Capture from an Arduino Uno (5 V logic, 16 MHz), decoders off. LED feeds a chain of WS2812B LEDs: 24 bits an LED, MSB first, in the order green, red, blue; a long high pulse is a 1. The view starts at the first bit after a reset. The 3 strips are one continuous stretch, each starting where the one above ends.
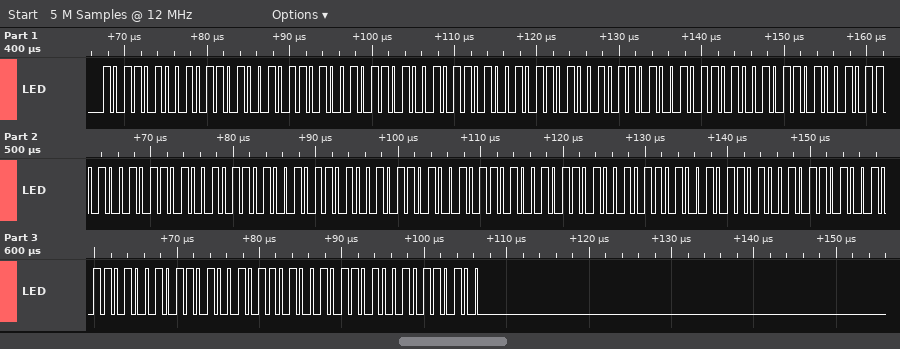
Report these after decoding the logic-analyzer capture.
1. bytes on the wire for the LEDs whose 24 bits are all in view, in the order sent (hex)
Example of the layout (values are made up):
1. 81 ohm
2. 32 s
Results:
1. B4 B4 B4 B4 B4 B4 B4 B4 B4 B4 B4 B4 B4 B4 B4 B4 B4 B4 B4 B4 B4 B4 B4 B4
